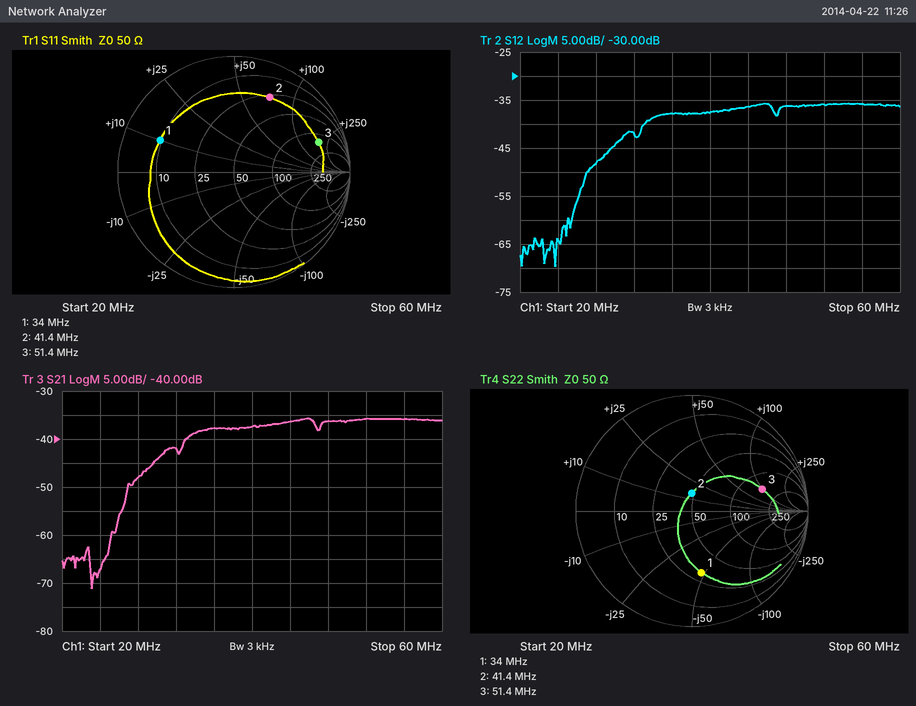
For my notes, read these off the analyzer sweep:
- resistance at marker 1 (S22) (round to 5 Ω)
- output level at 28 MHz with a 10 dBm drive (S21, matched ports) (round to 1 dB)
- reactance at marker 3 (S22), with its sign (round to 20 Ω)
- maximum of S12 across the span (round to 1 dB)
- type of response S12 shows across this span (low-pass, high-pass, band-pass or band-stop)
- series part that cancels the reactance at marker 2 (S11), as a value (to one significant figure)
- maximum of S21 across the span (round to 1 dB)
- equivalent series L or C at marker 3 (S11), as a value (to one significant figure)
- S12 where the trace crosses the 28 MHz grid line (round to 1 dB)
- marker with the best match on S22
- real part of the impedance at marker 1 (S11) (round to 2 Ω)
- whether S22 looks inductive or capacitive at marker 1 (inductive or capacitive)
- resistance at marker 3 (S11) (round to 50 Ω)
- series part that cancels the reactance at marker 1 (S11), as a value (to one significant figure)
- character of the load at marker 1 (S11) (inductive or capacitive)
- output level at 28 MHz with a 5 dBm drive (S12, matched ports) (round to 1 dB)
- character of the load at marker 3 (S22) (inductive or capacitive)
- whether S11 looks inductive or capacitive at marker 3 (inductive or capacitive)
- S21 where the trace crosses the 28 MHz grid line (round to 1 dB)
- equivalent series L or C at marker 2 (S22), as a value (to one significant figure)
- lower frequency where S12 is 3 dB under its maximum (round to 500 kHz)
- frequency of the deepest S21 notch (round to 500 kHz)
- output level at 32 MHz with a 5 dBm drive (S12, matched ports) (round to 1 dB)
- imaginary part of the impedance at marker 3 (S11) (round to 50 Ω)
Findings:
30 Ω
-38 dBm
+100 Ω
-36 dB
high-pass
50 pF
-36 dB
600 nH
-48 dB
marker 2
10 Ω
capacitive
150 Ω
500 pF
inductive
-43 dBm
inductive
inductive
-48 dB
60 nH
34.0 MHz
23.0 MHz
-37 dBm
+200 Ω
